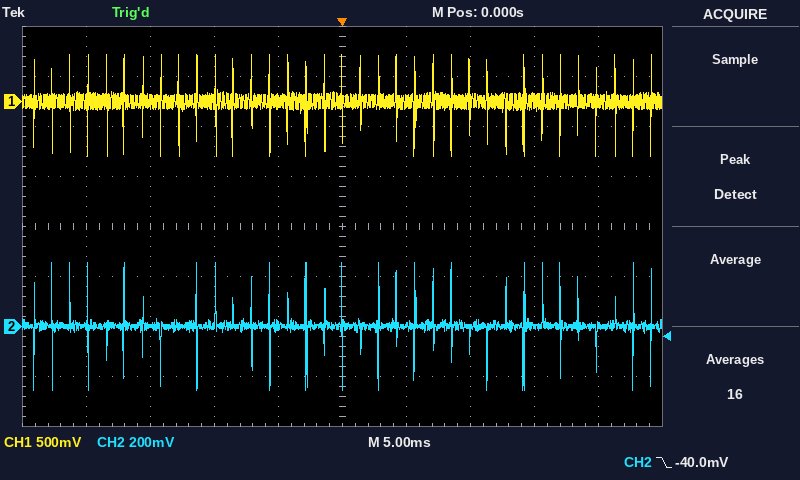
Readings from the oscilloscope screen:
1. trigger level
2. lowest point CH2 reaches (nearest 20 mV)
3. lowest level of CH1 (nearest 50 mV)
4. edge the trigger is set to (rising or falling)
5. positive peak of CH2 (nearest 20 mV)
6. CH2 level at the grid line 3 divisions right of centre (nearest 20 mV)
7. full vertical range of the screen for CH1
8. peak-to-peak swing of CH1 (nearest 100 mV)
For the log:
-40.0 mV
-260 mV
-550 mV
falling
260 mV
0 mV
4 V
1.00 V
